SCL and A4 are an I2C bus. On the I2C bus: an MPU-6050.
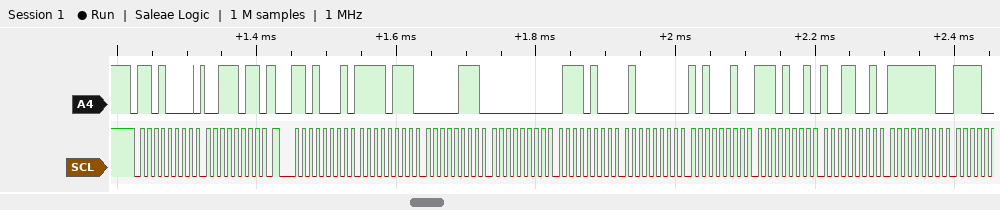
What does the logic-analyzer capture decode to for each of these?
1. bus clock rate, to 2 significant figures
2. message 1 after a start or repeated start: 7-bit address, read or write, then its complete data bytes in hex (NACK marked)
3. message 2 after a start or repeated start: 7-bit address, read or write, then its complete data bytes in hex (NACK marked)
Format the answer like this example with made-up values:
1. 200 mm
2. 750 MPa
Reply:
1. 100 kHz
2. 0x68 write: 3B
3. 0x68 read: F7 07 00 74 40 A2 E9 99 FE
